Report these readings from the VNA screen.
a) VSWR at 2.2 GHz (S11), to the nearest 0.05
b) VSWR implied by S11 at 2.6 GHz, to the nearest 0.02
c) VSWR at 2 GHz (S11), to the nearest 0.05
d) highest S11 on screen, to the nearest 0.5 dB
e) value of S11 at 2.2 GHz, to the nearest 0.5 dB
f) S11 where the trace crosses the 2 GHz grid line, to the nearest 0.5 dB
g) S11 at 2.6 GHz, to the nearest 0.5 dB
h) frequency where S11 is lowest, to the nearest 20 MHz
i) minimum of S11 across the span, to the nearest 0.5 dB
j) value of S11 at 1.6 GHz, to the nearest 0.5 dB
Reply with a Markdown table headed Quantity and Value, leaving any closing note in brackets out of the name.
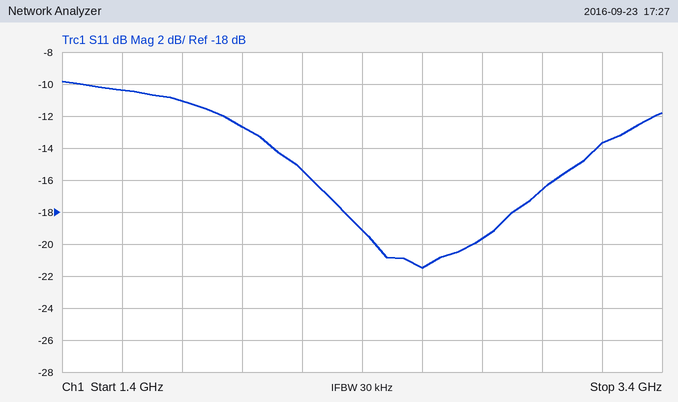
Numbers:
| Quantity | Value |
|---|---|
| VSWR at 2.2 GHz (S11), to the nearest 0.05 | 1.40 |
| VSWR implied by S11 at 2.6 GHz, to the nearest 0.02 | 1.18 |
| VSWR at 2 GHz (S11), to the nearest 0.05 | 1.60 |
| highest S11 on screen, to the nearest 0.5 dB | -10.0 dB |
| value of S11 at 2.2 GHz, to the nearest 0.5 dB | -15.5 dB |
| S11 where the trace crosses the 2 GHz grid line, to the nearest 0.5 dB | -12.5 dB |
| S11 at 2.6 GHz, to the nearest 0.5 dB | -21.5 dB |
| frequency where S11 is lowest, to the nearest 20 MHz | 2.60 GHz |
| minimum of S11 across the span, to the nearest 0.5 dB | -21.5 dB |
| value of S11 at 1.6 GHz, to the nearest 0.5 dB | -10.5 dB |
